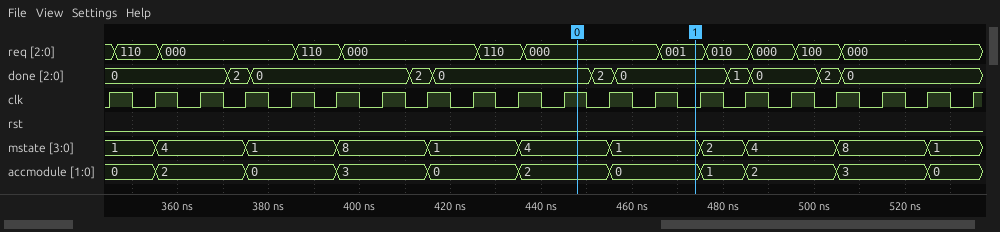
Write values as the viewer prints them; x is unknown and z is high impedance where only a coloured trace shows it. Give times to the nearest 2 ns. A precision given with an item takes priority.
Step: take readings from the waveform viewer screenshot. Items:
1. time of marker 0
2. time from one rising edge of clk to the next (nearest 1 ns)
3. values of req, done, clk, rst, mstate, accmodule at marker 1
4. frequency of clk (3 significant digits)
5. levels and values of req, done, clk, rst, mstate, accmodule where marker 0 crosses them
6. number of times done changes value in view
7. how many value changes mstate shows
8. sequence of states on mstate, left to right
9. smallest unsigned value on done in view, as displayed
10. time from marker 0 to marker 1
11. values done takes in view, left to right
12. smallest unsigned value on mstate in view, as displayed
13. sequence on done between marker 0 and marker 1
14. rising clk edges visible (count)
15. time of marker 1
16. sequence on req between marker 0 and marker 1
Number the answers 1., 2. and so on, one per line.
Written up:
1. 448 ns
2. 10 ns
3. req=001, done=0, clk=0, rst=0, mstate=1, accmodule=0
4. 100 MHz
5. req=000, done=0, clk=1, rst=0, mstate=4, accmodule=2
6. 10
7. 10
8. 1, 4, 1, 8, 1, 4, 1, 2, 4, 8, 1
9. 0
10. 26 ns
11. 0, 2, 0, 2, 0, 2, 0, 1, 0, 2, 0
12. 1
13. 0, 2, 0
14. 20
15. 474 ns
16. 000, 001
